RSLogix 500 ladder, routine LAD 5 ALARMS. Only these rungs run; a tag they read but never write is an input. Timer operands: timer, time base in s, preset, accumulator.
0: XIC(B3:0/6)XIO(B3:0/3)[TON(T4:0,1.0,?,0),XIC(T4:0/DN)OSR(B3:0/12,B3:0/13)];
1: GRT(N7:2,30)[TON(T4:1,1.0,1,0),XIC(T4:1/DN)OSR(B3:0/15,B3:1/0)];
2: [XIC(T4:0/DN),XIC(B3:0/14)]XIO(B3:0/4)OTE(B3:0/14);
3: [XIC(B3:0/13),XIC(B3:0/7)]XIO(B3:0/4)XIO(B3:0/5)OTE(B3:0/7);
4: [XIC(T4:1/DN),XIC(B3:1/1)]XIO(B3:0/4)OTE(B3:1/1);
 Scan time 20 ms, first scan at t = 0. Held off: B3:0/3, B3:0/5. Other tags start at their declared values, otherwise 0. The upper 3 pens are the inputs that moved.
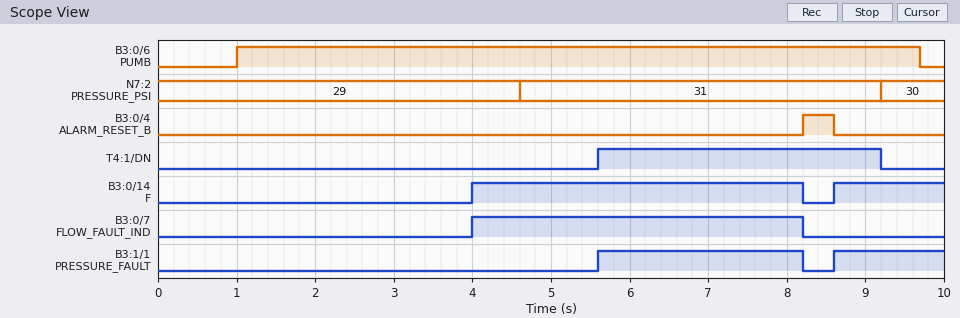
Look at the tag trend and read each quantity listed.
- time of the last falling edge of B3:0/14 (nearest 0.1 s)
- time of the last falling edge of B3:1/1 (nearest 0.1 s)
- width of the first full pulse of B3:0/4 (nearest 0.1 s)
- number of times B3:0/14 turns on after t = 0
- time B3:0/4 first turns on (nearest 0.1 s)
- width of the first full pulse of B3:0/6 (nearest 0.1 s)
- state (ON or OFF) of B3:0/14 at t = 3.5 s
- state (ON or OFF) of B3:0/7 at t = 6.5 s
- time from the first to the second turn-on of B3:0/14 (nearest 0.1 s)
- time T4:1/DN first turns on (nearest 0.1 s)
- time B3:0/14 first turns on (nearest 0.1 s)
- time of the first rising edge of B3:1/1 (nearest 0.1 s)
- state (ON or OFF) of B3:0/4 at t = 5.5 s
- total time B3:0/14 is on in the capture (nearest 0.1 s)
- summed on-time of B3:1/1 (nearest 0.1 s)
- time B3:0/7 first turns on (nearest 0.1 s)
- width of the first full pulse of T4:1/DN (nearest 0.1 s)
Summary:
8.2 s
8.2 s
0.4 s
2
8.2 s
8.7 s
OFF
ON
4.6 s
5.6 s
4.0 s
5.6 s
OFF
5.6 s
4.0 s
4.0 s
3.6 s
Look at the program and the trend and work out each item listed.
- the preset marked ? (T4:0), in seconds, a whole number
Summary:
3 s
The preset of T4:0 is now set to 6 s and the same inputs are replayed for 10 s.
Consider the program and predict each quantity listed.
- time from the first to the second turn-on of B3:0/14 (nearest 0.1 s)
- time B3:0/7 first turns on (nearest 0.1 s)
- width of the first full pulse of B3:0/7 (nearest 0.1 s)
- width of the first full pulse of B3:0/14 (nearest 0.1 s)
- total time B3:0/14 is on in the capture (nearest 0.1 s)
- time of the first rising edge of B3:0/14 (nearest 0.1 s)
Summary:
1.6 s
7.0 s
1.2 s
1.2 s
2.6 s
7.0 s
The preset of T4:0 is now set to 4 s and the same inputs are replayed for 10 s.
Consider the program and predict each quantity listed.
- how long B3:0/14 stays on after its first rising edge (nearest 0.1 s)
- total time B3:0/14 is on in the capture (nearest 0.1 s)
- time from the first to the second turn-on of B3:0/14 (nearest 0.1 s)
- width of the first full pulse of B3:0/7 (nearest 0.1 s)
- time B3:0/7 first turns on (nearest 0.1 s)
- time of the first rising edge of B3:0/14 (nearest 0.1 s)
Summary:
3.2 s
4.6 s
3.6 s
3.2 s
5.0 s
5.0 s
